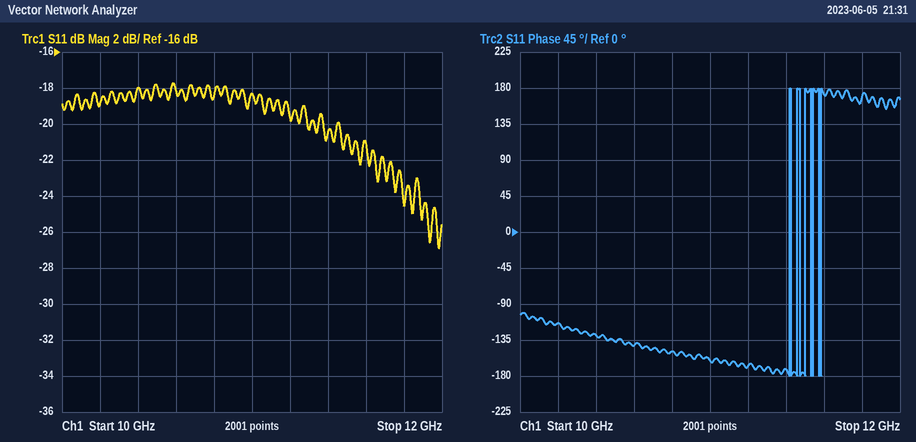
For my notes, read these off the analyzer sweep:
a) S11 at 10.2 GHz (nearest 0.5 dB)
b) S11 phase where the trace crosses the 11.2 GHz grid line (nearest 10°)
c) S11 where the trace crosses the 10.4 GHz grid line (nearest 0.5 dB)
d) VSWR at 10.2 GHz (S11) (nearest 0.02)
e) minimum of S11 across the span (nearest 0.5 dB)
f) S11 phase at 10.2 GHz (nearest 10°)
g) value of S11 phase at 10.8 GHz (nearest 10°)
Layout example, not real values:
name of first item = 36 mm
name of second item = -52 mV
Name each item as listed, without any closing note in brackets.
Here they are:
S11 at 10.2 GHz = -19.0 dB
S11 phase where the trace crosses the 11.2 GHz grid line = -170°
S11 where the trace crosses the 10.4 GHz grid line = -18.0 dB
VSWR at 10.2 GHz (S11) = 1.26
minimum of S11 across the span = -27.0 dB
S11 phase at 10.2 GHz = -110°
value of S11 phase at 10.8 GHz = -150°
